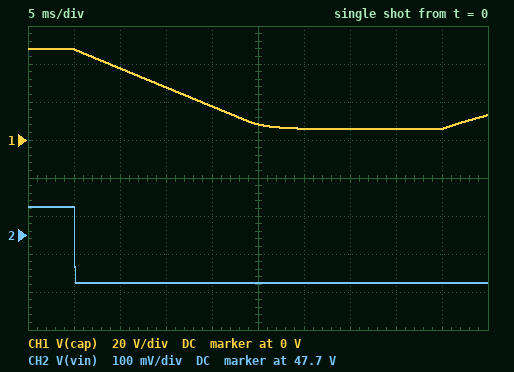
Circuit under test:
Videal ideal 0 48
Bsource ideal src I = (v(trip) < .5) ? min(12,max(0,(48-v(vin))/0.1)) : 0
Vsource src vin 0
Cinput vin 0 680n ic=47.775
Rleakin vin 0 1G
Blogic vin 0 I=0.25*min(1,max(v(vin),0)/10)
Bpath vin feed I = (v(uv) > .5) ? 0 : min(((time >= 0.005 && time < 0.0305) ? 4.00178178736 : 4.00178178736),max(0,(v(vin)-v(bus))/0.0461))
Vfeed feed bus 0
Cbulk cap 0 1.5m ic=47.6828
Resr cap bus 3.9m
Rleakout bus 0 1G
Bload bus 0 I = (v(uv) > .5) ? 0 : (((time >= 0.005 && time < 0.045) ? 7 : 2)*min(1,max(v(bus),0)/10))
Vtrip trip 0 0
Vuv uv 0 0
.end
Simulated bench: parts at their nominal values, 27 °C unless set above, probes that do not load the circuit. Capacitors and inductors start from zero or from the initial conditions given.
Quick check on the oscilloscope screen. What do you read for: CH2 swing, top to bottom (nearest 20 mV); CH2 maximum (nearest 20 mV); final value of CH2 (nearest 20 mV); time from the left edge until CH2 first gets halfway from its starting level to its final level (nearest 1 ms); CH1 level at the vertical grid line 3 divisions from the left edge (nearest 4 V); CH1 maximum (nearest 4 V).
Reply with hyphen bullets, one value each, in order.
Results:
- 200 mV
- 47.78 V
- 47.58 V
- 5 ms
- 28 V
- 48 V
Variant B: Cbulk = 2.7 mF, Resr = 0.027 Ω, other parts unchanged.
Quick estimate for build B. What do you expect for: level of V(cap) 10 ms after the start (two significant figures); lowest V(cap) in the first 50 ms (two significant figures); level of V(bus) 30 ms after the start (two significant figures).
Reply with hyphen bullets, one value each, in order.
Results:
- 42 V
- 6.6 V
- 20 V
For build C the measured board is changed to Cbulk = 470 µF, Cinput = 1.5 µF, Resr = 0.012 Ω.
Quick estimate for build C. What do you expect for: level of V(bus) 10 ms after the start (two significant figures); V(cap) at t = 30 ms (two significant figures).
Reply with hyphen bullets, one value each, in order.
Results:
- 16 V
- 5.7 V
